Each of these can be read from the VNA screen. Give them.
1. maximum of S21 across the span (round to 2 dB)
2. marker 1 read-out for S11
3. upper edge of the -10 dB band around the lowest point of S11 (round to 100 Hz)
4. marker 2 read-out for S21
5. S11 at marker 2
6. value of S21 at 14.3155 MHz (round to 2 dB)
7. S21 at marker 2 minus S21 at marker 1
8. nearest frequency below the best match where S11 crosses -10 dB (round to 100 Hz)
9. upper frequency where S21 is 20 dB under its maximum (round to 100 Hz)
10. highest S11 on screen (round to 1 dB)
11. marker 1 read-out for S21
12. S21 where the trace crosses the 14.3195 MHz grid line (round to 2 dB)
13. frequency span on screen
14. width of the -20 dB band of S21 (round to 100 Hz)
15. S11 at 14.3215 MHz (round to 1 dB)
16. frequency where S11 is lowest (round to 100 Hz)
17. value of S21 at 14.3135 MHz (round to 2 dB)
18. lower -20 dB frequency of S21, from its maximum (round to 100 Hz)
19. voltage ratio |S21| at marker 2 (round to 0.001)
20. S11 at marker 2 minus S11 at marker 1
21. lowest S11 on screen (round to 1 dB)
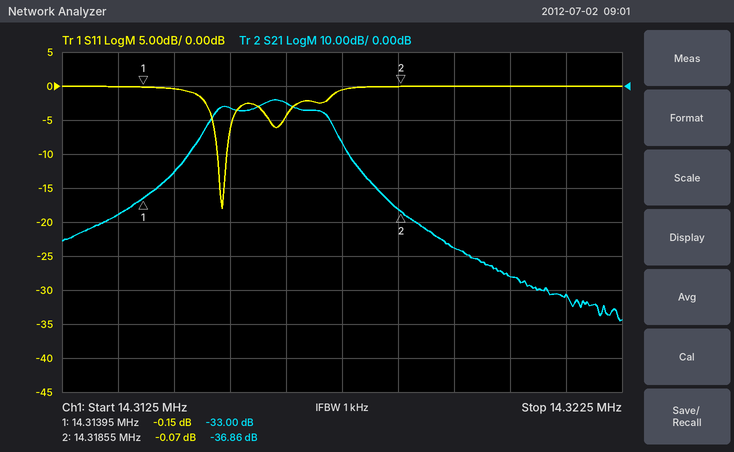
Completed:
-4 dB
-0.15 dB
14.3154 MHz
-36.86 dB
-0.07 dB
-6 dB
-3.86 dB
14.3153 MHz
14.3178 MHz
0 dB
-33.00 dB
-48 dB
10 kHz
3.2 kHz
0 dB
14.3154 MHz
-38 dB
14.3146 MHz
0.014
0.08 dB
-18 dB
